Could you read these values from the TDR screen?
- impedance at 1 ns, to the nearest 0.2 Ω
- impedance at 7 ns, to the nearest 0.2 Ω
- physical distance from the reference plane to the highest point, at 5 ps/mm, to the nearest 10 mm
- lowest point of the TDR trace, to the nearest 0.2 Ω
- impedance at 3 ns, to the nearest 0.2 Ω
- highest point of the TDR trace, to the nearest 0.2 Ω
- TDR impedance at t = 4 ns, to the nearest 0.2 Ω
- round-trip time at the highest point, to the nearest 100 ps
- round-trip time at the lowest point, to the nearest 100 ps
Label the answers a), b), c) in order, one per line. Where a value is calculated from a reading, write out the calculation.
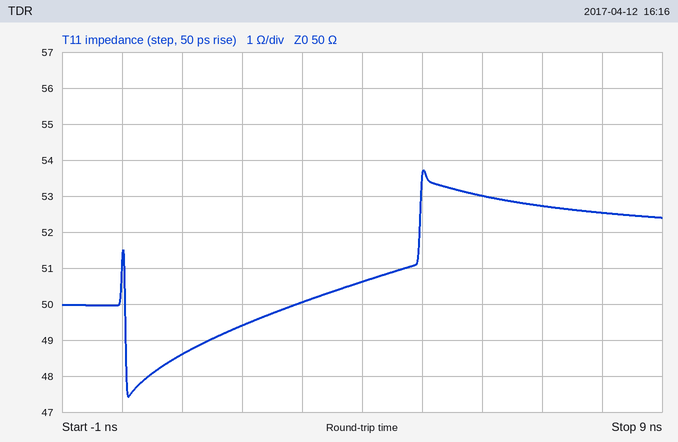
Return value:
a) 48.6 Ω
b) 52.8 Ω
c) 5.0 ns / 2 / 5 ps/mm ≈ 500 mm
d) 47.4 Ω
e) 50.0 Ω
f) 53.8 Ω
g) 50.6 Ω
h) 5.0 ns
i) 100 ps
